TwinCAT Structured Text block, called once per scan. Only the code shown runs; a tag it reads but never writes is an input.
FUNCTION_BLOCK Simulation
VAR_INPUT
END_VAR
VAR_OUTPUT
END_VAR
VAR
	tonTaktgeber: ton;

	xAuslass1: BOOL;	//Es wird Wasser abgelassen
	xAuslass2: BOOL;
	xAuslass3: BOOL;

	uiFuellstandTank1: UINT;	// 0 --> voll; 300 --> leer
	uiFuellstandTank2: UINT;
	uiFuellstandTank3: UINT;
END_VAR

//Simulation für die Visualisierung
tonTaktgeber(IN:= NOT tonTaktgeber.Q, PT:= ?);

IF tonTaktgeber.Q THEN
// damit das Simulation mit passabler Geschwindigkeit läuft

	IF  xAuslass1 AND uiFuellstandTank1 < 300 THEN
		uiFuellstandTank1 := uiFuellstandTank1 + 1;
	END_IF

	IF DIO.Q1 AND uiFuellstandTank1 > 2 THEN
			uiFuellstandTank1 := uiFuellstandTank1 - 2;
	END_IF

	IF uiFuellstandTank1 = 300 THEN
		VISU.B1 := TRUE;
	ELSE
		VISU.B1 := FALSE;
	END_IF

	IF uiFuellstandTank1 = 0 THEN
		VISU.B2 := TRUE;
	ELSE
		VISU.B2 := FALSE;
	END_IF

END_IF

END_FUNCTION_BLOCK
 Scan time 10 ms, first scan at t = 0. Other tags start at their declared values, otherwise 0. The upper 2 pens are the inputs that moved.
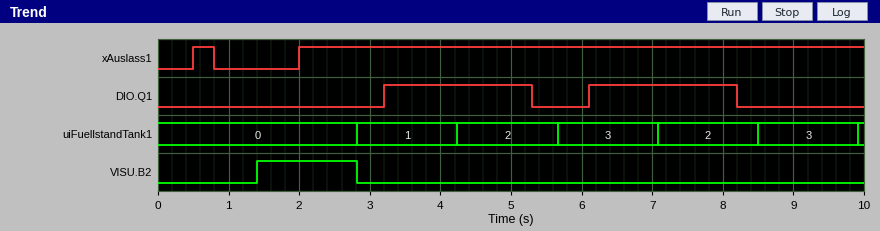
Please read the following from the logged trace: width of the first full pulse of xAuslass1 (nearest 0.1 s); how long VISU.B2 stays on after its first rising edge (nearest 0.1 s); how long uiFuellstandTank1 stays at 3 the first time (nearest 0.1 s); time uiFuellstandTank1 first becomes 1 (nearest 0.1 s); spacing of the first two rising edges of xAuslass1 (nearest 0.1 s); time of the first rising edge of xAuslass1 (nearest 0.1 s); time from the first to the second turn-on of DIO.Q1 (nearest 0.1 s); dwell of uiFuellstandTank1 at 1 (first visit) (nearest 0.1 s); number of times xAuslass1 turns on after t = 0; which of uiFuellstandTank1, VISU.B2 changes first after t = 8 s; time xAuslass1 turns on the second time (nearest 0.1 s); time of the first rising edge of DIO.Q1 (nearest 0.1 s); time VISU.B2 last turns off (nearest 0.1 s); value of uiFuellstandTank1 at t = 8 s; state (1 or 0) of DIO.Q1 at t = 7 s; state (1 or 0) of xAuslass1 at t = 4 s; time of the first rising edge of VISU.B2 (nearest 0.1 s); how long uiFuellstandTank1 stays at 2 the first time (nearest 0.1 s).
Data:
0.3 s
1.4 s
1.4 s
2.8 s
1.5 s
0.5 s
2.9 s
1.4 s
2
uiFuellstandTank1
2.0 s
3.2 s
2.8 s
2
1
1
1.4 s
1.4 s
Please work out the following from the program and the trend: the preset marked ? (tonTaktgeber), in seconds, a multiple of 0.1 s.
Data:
1.4 s
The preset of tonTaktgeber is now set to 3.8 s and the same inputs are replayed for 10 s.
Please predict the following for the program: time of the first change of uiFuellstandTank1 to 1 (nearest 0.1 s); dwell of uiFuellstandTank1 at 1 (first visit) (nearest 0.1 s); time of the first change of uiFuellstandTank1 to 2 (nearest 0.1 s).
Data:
3.8 s
3.8 s
7.6 s
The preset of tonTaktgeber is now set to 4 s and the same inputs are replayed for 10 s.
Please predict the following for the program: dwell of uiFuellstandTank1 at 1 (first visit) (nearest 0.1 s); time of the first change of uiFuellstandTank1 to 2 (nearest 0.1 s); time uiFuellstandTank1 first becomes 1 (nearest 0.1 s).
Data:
4.0 s
8.0 s
4.0 s
